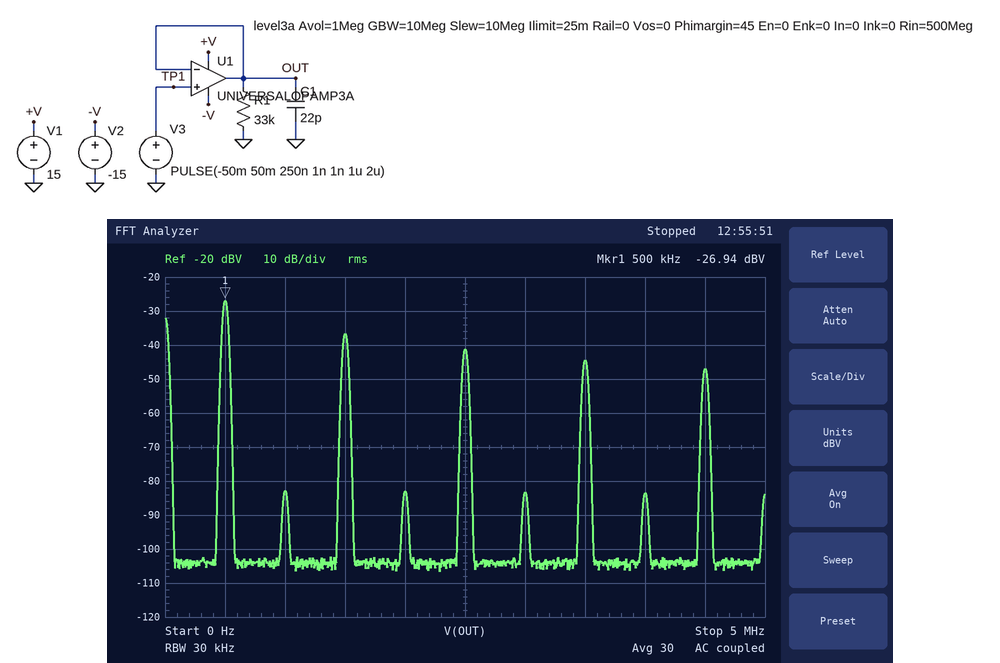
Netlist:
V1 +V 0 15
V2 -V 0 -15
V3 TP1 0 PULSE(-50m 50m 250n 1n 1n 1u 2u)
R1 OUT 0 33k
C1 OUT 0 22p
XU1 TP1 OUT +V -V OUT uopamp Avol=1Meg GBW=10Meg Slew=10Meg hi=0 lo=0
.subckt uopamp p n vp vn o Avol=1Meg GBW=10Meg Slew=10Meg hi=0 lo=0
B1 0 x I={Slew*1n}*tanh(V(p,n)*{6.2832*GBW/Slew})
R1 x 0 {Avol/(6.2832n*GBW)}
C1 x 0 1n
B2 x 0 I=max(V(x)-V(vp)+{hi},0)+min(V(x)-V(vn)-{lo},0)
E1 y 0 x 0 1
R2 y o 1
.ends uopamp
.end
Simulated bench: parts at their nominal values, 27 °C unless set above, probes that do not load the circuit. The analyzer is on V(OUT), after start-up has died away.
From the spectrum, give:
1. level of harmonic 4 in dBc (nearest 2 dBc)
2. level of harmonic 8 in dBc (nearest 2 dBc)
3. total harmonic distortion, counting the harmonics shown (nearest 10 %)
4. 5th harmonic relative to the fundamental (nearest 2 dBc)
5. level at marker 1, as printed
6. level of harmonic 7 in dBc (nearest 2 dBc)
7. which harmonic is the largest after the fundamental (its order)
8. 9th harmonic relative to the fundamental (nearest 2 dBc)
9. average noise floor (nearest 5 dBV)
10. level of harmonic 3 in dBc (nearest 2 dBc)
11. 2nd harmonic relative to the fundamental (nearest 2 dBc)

-56 dBc
-56 dBc
40 %
-14 dBc
-26.94 dBV
-18 dBc
3
-20 dBc
-105 dBV
-10 dBc
-56 dBc
